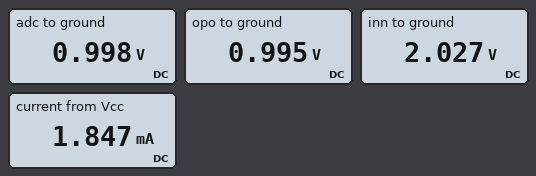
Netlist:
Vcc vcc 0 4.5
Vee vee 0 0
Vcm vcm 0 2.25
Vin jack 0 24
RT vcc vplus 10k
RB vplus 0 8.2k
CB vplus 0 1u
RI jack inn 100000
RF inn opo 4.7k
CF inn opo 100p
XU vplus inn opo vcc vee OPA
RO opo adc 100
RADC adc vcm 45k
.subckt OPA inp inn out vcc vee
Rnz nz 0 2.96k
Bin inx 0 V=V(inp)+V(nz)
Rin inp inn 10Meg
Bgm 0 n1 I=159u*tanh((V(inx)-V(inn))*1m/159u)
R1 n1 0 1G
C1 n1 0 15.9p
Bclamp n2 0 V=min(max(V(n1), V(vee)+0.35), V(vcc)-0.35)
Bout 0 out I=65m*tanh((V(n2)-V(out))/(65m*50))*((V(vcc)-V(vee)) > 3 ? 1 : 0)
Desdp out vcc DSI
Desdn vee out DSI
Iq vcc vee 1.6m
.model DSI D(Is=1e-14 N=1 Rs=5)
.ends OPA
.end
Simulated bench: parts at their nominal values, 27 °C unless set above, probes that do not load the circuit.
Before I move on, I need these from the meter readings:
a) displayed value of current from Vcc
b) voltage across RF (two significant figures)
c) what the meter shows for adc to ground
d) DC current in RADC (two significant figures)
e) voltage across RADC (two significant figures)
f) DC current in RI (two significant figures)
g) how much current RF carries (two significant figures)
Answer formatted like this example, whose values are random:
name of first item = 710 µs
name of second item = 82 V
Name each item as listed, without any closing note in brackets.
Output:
displayed value of current from Vcc = 1.847 mA
voltage across RF = 1.0 V
what the meter shows for adc to ground = 0.998 V
DC current in RADC = 28 µA
voltage across RADC = 1.3 V
DC current in RI = 220 µA
how much current RF carries = 220 µA
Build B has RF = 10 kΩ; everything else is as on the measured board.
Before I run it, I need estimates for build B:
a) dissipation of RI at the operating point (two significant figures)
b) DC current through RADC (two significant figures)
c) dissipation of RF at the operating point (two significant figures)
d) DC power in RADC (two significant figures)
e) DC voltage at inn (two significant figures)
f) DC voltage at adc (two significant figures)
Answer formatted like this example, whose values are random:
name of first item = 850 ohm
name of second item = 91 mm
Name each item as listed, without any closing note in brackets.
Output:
dissipation of RI at the operating point = 4.6 mW
DC current through RADC = 42 µA
dissipation of RF at the operating point = 460 µW
DC power in RADC = 79 µW
DC voltage at inn = 2.5 V
DC voltage at adc = 370 mV
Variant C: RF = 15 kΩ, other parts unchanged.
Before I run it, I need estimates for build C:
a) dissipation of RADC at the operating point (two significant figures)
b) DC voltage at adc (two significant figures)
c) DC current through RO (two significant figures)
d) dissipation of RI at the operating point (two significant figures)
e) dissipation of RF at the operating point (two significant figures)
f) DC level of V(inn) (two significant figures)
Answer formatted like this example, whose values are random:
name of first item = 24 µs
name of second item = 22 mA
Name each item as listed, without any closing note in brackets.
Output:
dissipation of RADC at the operating point = 79 µW
DC voltage at adc = 370 mV
DC current through RO = 42 µA
dissipation of RI at the operating point = 4.2 mW
dissipation of RF at the operating point = 630 µW
DC level of V(inn) = 3.4 V
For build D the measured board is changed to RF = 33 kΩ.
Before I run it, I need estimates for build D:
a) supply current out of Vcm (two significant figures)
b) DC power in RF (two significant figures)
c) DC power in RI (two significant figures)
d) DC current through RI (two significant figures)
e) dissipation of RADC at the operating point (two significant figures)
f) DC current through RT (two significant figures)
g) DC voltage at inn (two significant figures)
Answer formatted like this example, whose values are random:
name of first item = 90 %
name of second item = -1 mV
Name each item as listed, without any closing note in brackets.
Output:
supply current out of Vcm = 42 µA
DC power in RF = 1.0 mW
DC power in RI = 3.2 mW
DC current through RI = 180 µA
dissipation of RADC at the operating point = 79 µW
DC current through RT = 250 µA
DC voltage at inn = 6.2 V
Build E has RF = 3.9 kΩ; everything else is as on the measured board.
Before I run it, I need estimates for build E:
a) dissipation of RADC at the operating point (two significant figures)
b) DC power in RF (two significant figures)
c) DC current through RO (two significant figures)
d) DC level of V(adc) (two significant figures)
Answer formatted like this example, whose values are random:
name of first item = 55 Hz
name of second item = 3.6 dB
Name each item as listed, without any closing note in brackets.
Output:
dissipation of RADC at the operating point = 26 µW
DC power in RF = 190 µW
DC current through RO = 24 µA
DC level of V(adc) = 1.2 V
